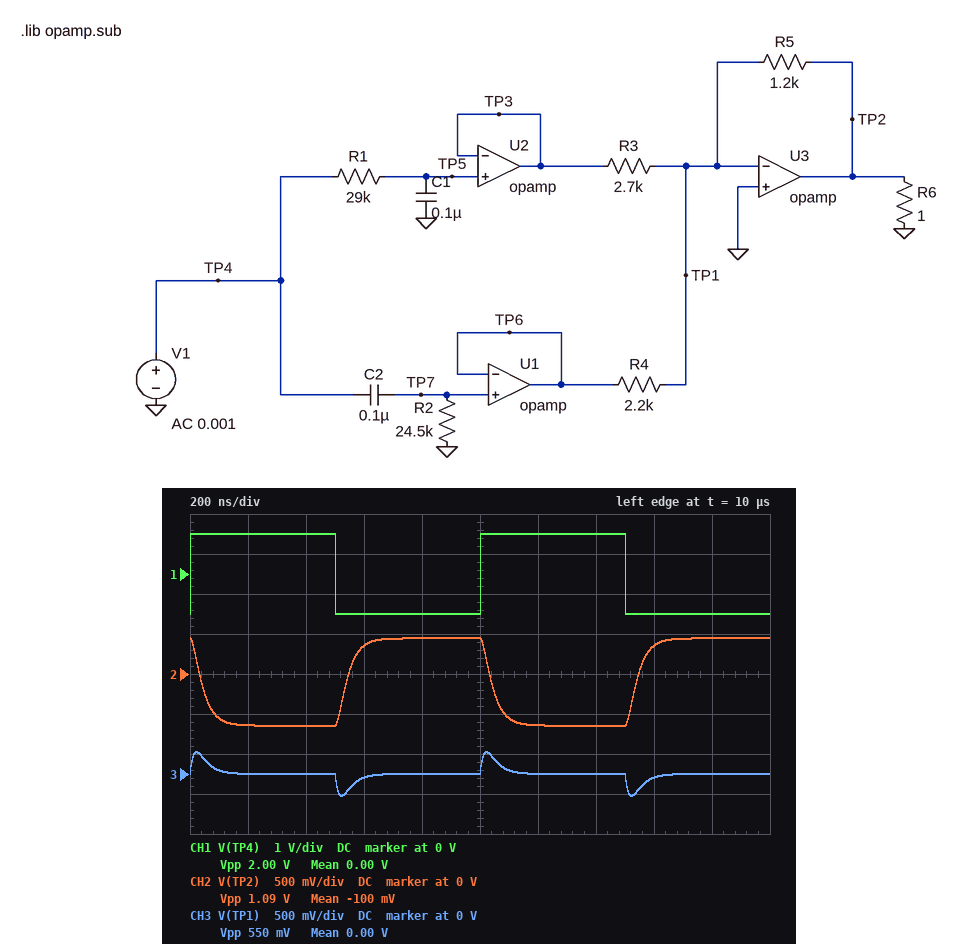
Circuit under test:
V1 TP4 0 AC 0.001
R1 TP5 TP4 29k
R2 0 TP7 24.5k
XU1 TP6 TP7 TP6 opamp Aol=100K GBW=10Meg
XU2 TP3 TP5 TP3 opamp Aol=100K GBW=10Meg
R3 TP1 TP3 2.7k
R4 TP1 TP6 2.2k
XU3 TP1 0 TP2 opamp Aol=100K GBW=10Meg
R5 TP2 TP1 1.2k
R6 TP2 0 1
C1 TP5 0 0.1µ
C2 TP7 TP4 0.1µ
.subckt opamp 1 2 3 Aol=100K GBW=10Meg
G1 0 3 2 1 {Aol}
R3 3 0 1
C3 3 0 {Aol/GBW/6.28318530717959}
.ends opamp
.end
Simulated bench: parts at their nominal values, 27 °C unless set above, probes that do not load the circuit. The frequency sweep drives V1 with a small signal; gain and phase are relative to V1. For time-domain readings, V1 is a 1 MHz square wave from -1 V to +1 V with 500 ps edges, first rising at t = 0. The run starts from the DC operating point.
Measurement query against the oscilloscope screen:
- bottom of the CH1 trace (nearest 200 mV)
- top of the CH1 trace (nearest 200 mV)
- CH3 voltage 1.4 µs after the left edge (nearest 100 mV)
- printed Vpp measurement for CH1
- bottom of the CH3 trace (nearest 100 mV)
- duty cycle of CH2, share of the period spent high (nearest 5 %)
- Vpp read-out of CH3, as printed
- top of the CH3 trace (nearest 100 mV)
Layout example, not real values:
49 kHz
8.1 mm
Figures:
-1.0 V
1.0 V
0 V
2.00 V
-300 mV
50 %
550 mV
300 mV
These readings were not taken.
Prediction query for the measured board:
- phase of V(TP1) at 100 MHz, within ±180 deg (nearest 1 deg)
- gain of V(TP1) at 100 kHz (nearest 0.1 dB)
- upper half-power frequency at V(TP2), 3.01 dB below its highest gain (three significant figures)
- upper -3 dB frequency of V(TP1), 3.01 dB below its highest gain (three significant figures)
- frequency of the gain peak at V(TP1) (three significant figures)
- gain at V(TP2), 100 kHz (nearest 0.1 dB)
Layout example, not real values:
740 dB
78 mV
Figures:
-81 deg
-45.3 dB
4.20 MHz
17.8 MHz
7.09 MHz
-5.3 dB
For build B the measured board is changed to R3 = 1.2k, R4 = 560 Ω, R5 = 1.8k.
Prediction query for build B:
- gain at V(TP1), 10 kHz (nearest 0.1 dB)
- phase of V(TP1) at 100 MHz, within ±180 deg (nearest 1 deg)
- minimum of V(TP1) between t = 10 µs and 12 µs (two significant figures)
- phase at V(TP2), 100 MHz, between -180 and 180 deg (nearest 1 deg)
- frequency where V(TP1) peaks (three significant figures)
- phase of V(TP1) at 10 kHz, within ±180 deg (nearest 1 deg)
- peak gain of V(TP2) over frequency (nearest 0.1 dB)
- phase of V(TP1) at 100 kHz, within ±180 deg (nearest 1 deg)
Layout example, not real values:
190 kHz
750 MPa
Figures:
-49.9 dB
-83 deg
-770 mV
7 deg
4.18 MHz
89 deg
10.1 dB
86 deg
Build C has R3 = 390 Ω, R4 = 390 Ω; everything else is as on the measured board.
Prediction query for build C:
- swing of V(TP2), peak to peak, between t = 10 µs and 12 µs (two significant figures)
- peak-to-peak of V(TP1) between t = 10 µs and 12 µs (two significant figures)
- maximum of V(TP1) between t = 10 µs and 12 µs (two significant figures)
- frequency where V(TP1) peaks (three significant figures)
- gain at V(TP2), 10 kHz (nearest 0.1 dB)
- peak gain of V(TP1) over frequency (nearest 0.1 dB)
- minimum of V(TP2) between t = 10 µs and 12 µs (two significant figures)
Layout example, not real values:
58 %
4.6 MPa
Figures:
6.0 V
1.2 V
620 mV
3.74 MHz
9.8 dB
-8.5 dB
-3.0 V
